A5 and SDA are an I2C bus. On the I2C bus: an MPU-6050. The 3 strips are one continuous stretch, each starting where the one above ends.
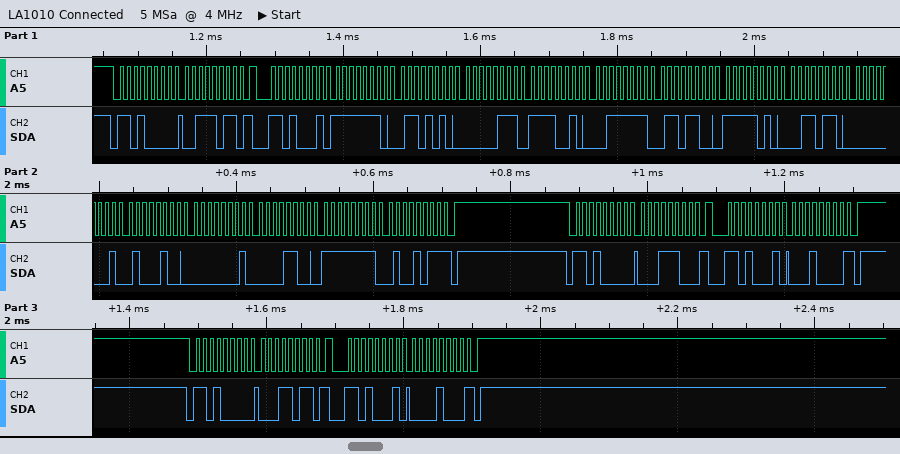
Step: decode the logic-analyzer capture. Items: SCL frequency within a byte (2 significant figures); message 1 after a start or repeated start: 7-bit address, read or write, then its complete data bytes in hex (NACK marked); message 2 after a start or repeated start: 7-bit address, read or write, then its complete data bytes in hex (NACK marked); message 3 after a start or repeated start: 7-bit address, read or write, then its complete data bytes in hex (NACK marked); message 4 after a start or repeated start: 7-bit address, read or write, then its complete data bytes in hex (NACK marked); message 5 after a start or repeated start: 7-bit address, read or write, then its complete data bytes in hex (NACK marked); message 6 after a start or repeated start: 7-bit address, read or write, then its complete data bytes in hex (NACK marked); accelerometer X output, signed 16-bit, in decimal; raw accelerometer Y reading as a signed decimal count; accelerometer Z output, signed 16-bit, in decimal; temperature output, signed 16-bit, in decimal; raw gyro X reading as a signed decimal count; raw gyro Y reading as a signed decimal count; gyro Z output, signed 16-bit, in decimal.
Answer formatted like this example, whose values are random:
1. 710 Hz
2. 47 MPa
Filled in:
1. 100 kHz
2. 0x68 write: 3B
3. 0x68 read: FE 6A 07 F2 3F 6C FA 36 01 44 01 0C FF 4B NACK
4. 0x68 write: 1C
5. 0x68 read: 10 NACK
6. 0x68 write: 1B
7. 0x68 read: 08 NACK
8. -406
9. 2034
10. 16236
11. -1482
12. 324
13. 268
14. -181
